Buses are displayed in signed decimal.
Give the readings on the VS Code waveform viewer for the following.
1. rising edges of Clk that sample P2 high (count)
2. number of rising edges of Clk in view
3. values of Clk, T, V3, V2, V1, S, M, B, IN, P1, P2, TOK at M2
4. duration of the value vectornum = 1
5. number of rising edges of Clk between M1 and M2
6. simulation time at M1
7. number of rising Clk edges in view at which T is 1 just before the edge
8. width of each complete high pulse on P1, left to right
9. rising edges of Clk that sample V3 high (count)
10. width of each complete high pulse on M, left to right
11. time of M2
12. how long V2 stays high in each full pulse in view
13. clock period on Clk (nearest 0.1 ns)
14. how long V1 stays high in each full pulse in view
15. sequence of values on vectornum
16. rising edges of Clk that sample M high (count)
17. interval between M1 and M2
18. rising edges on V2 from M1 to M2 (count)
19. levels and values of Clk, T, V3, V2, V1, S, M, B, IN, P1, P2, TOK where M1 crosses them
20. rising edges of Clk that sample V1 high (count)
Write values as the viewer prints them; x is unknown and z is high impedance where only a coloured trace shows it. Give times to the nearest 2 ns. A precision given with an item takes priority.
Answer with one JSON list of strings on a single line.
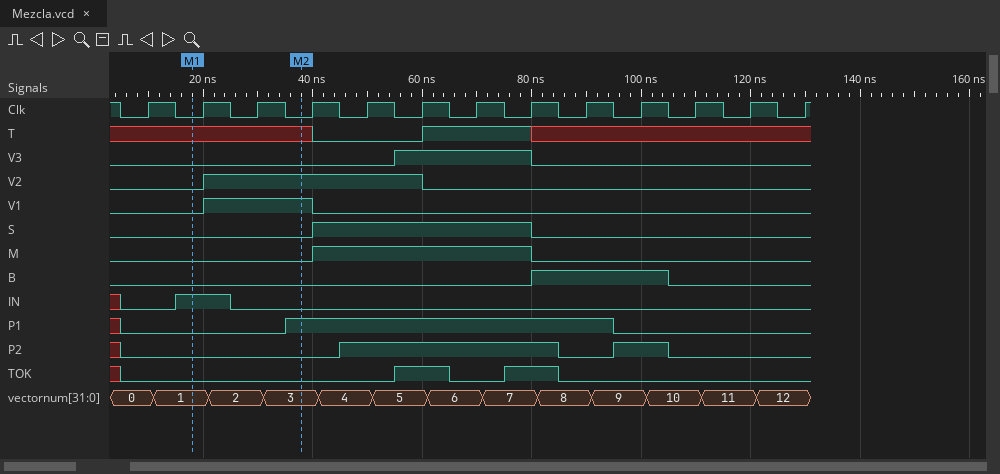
["5", "13", "Clk=0, T=x, V3=0, V2=1, V1=1, S=0, M=0, B=0, IN=0, P1=1, P2=0, TOK=0", "10 ns", "2", "18 ns", "2", "60 ns", "3", "40 ns", "38 ns", "40 ns", "10 ns", "20 ns", "0, 1, 2, 3, 4, 5, 6, 7, 8, 9, 10, 11, 12", "4", "20 ns", "1", "Clk=0, T=x, V3=0, V2=0, V1=0, S=0, M=0, B=0, IN=1, P1=0, P2=0, TOK=0", "2"]
